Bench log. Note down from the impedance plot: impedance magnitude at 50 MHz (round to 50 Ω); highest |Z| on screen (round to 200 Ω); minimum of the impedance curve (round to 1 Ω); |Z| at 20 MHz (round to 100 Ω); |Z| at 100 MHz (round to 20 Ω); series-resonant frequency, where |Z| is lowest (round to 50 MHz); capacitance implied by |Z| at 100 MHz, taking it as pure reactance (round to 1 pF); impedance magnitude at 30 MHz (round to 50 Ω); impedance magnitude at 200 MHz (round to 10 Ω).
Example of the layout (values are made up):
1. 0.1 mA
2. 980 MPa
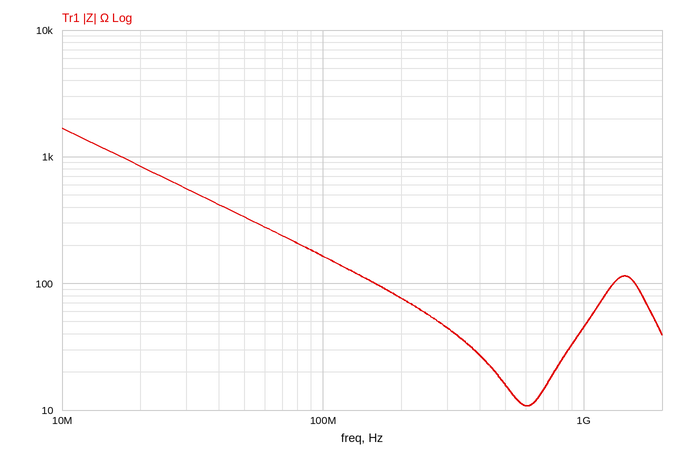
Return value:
1. 350 Ω
2. 1.6 kΩ
3. 11 Ω
4. 800 Ω
5. 160 Ω
6. 600 MHz
7. 10 pF
8. 550 Ω
9. 80 Ω
